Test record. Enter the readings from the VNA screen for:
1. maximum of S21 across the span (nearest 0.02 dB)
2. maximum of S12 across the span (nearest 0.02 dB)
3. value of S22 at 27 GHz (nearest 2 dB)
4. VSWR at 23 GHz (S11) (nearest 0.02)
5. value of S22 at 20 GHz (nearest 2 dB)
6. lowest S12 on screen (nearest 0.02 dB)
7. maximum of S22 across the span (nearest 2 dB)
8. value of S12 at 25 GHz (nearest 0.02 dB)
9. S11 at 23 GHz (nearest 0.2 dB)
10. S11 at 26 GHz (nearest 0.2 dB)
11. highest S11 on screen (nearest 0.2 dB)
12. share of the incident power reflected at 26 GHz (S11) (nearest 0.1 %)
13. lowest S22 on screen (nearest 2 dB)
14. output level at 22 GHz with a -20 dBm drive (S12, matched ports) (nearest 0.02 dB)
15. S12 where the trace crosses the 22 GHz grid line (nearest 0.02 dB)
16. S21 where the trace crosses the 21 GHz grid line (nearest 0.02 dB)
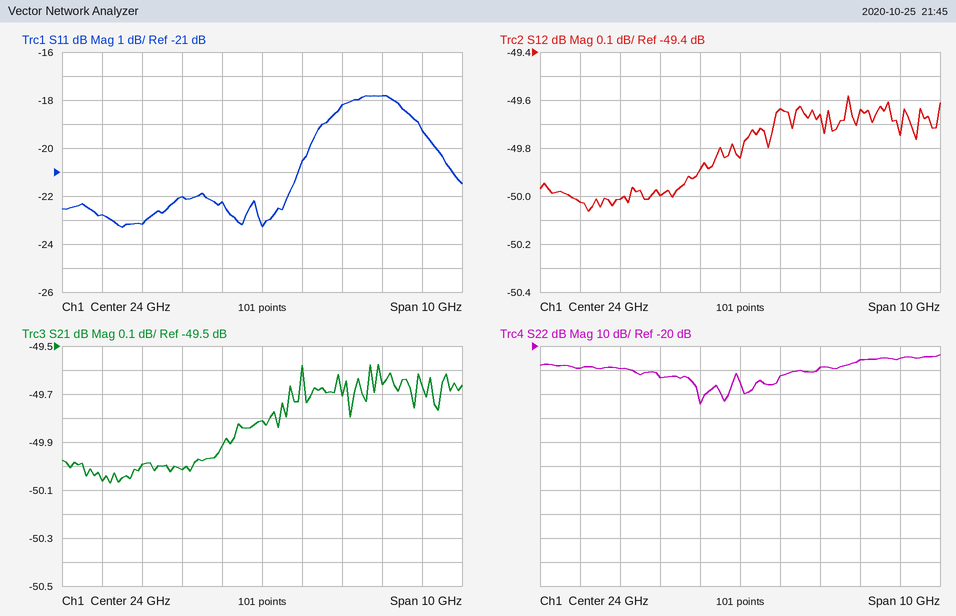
-49.58 dB
-49.58 dB
-26 dB
1.16
-30 dB
-50.06 dB
-24 dB
-49.64 dB
-22.2 dB
-18.2 dB
-17.8 dB
1.5 %
-44 dB
-70.00 dBm
-50.00 dB
-50.00 dB
